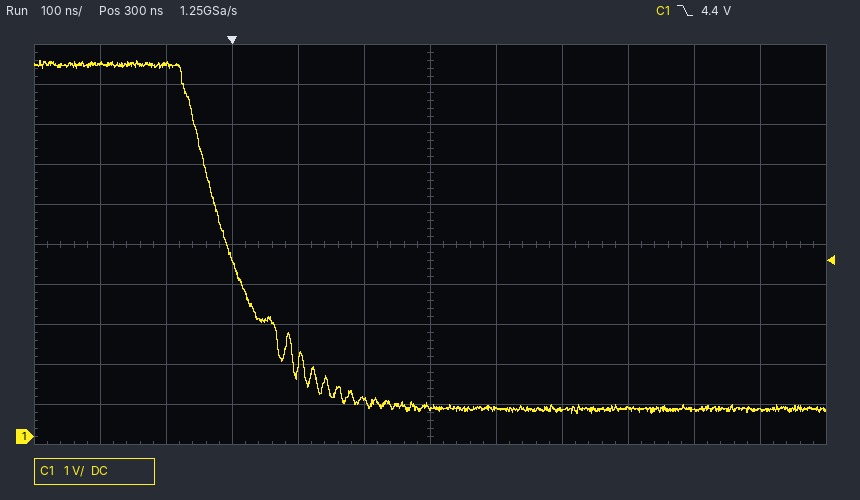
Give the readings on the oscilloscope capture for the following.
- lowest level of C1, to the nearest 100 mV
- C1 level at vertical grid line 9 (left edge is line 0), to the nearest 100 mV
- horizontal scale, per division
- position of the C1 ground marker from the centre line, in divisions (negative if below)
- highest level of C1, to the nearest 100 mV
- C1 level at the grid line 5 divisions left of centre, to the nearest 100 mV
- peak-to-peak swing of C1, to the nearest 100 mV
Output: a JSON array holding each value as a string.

["600 mV", "700 mV", "100 ns", "-4.8 div", "9.4 V", "9.3 V", "8.8 V"]
